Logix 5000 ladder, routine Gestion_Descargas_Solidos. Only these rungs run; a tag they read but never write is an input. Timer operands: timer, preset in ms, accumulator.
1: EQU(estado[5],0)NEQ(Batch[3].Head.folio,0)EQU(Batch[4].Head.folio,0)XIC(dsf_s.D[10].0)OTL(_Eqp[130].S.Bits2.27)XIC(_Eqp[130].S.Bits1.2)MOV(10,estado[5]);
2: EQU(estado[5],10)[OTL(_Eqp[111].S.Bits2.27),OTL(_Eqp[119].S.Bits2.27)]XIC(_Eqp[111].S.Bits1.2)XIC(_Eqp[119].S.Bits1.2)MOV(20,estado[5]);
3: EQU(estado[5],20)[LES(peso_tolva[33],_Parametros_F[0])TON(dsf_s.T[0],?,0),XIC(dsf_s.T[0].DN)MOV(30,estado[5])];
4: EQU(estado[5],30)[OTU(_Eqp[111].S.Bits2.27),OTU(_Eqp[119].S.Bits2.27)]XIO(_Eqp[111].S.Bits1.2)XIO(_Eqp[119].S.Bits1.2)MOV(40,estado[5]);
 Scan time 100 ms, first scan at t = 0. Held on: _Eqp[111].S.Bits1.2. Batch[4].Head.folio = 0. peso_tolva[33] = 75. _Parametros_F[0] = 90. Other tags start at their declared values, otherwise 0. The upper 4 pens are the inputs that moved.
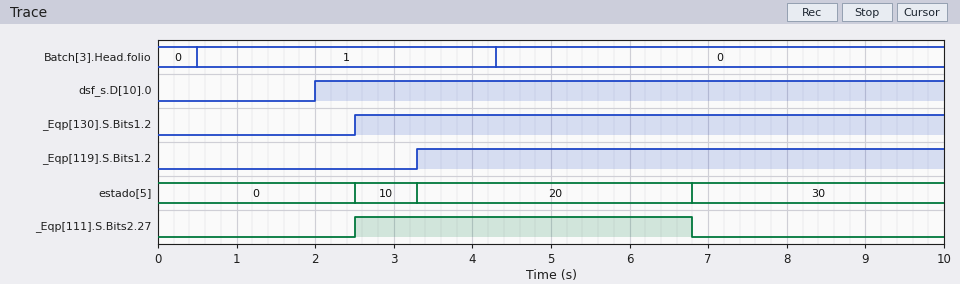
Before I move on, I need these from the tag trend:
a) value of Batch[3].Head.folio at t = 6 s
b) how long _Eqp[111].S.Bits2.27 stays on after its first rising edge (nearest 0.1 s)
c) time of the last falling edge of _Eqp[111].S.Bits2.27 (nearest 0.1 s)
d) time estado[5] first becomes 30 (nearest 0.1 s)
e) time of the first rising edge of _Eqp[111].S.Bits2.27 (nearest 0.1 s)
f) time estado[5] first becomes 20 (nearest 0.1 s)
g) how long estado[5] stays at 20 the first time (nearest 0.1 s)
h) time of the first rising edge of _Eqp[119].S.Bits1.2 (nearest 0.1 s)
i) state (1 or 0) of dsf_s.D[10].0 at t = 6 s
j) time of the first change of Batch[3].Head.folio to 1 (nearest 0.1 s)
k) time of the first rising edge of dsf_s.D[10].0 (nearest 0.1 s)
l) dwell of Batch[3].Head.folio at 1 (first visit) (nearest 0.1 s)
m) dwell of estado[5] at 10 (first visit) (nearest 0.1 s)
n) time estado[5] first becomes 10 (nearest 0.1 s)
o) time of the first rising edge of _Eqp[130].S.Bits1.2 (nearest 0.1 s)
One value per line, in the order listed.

0
4.3 s
6.8 s
6.8 s
2.5 s
3.3 s
3.5 s
3.3 s
1
0.5 s
2.0 s
3.8 s
0.8 s
2.5 s
2.5 s
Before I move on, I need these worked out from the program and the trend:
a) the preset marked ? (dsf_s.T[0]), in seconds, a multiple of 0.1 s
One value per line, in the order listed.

3.5 s
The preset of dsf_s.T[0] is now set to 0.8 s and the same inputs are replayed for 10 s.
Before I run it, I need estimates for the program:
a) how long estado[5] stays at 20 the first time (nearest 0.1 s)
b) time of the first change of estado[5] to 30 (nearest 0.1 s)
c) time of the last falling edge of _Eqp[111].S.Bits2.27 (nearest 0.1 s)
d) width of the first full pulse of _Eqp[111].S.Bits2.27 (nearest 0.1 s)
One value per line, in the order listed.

0.8 s
4.1 s
4.1 s
1.6 s
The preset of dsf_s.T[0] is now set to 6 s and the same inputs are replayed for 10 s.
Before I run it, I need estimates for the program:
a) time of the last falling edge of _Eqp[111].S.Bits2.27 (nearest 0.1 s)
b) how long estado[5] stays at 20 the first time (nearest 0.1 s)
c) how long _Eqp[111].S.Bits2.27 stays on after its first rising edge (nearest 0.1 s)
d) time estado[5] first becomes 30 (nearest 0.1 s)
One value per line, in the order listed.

9.3 s
6.0 s
6.8 s
9.3 s
